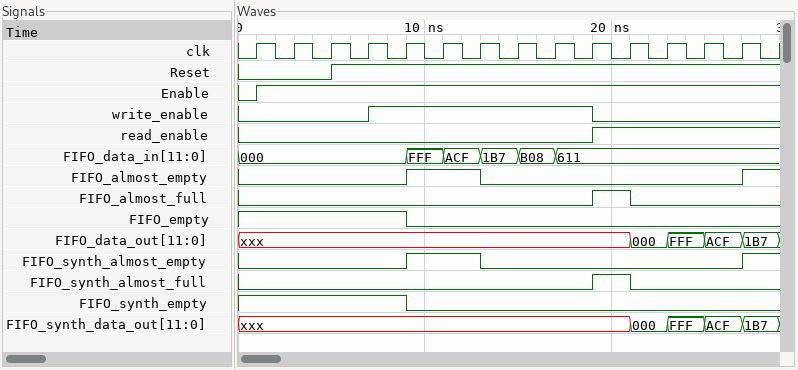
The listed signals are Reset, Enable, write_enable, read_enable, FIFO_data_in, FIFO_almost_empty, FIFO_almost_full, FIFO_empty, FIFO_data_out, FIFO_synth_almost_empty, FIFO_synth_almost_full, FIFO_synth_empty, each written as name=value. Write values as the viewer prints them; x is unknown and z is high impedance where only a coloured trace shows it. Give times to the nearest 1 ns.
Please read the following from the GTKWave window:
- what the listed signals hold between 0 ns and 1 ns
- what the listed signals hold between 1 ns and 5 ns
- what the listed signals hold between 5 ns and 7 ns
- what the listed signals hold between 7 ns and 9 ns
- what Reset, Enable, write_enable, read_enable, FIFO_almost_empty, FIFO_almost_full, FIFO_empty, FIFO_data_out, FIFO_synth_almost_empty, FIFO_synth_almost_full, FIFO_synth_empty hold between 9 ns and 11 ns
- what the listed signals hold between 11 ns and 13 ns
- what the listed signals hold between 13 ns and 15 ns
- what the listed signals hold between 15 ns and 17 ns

Reset=0, Enable=0, write_enable=0, read_enable=0, FIFO_data_in=000, FIFO_almost_empty=0, FIFO_almost_full=0, FIFO_empty=1, FIFO_data_out=xxx, FIFO_synth_almost_empty=0, FIFO_synth_almost_full=0, FIFO_synth_empty=1
Reset=0, Enable=1, write_enable=0, read_enable=0, FIFO_data_in=000, FIFO_almost_empty=0, FIFO_almost_full=0, FIFO_empty=1, FIFO_data_out=xxx, FIFO_synth_almost_empty=0, FIFO_synth_almost_full=0, FIFO_synth_empty=1
Reset=1, Enable=1, write_enable=0, read_enable=0, FIFO_data_in=000, FIFO_almost_empty=0, FIFO_almost_full=0, FIFO_empty=1, FIFO_data_out=xxx, FIFO_synth_almost_empty=0, FIFO_synth_almost_full=0, FIFO_synth_empty=1
Reset=1, Enable=1, write_enable=1, read_enable=0, FIFO_data_in=000, FIFO_almost_empty=0, FIFO_almost_full=0, FIFO_empty=1, FIFO_data_out=xxx, FIFO_synth_almost_empty=0, FIFO_synth_almost_full=0, FIFO_synth_empty=1
Reset=1, Enable=1, write_enable=1, read_enable=0, FIFO_almost_empty=1, FIFO_almost_full=0, FIFO_empty=0, FIFO_data_out=xxx, FIFO_synth_almost_empty=1, FIFO_synth_almost_full=0, FIFO_synth_empty=0
Reset=1, Enable=1, write_enable=1, read_enable=0, FIFO_data_in=ACF, FIFO_almost_empty=1, FIFO_almost_full=0, FIFO_empty=0, FIFO_data_out=xxx, FIFO_synth_almost_empty=1, FIFO_synth_almost_full=0, FIFO_synth_empty=0
Reset=1, Enable=1, write_enable=1, read_enable=0, FIFO_data_in=1B7, FIFO_almost_empty=0, FIFO_almost_full=0, FIFO_empty=0, FIFO_data_out=xxx, FIFO_synth_almost_empty=0, FIFO_synth_almost_full=0, FIFO_synth_empty=0
Reset=1, Enable=1, write_enable=1, read_enable=0, FIFO_data_in=B08, FIFO_almost_empty=0, FIFO_almost_full=0, FIFO_empty=0, FIFO_data_out=xxx, FIFO_synth_almost_empty=0, FIFO_synth_almost_full=0, FIFO_synth_empty=0
